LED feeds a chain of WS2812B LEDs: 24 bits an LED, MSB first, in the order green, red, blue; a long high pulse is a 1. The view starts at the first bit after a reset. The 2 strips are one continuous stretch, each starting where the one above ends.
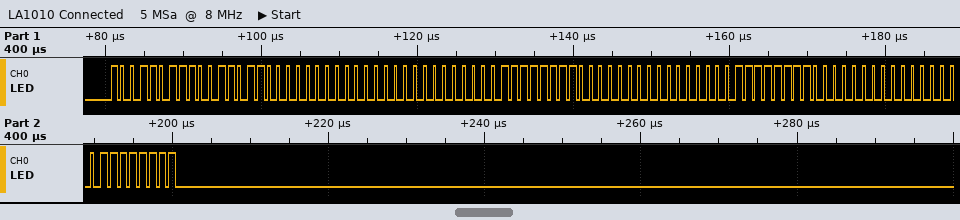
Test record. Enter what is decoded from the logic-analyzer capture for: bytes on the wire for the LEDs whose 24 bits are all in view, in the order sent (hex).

9B 9B 00 00 00 FF 00 00 FF 00 00 FF
